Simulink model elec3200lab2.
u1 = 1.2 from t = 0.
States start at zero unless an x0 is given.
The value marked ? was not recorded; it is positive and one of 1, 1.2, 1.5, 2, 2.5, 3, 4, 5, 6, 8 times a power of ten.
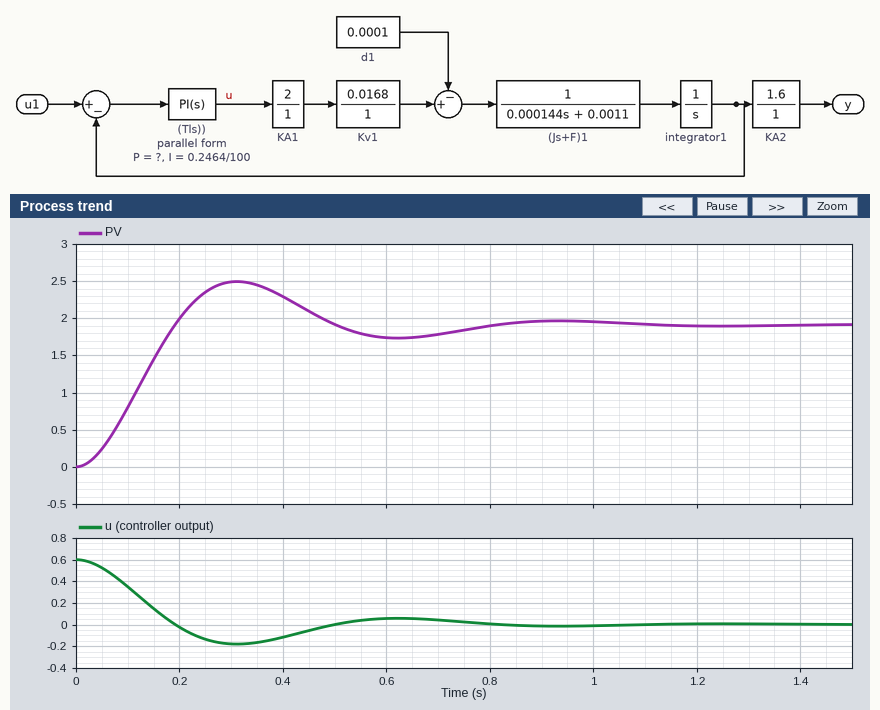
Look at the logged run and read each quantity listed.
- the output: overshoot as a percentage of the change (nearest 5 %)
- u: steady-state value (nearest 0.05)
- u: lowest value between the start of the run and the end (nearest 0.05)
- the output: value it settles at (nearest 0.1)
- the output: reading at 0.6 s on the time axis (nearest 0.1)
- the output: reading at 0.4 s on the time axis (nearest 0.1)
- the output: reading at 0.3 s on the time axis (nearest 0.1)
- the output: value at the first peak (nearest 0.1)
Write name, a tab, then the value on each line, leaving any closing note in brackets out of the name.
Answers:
the output: overshoot as a percentage of the change	30 %
u: steady-state value	0.00
u: lowest value between the start of the run and the end	-0.20
the output: value it settles at	1.9
the output: reading at 0.6 s on the time axis	1.7
the output: reading at 0.4 s on the time axis	2.3
the output: reading at 0.3 s on the time axis	2.5
the output: value at the first peak	2.5
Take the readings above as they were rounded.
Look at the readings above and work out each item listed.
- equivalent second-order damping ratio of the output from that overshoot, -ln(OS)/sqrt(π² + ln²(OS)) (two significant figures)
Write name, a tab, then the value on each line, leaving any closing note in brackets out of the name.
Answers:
equivalent second-order damping ratio of the output from that overshoot, -ln(OS)/sqrt(π² + ln²(OS))	0.36
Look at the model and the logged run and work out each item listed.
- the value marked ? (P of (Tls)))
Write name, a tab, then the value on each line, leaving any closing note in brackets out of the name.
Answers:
the value marked ? (P of (Tls)))	0.5
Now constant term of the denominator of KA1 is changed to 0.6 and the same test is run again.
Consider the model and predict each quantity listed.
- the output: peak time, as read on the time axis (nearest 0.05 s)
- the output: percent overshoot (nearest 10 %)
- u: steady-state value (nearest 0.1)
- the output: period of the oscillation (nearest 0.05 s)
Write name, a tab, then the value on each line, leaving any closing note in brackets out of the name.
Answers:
the output: peak time, as read on the time axis	0.25 s
the output: percent overshoot	40 %
u: steady-state value	0.0
the output: period of the oscillation	0.45 s
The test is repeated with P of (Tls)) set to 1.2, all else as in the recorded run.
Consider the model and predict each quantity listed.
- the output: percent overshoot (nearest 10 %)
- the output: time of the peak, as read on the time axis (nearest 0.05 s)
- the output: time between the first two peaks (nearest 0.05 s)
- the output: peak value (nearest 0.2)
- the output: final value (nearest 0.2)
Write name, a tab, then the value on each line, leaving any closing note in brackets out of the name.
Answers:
the output: percent overshoot	50 %
the output: time of the peak, as read on the time axis	0.20 s
the output: time between the first two peaks	0.40 s
the output: peak value	2.8
the output: final value	2.0
